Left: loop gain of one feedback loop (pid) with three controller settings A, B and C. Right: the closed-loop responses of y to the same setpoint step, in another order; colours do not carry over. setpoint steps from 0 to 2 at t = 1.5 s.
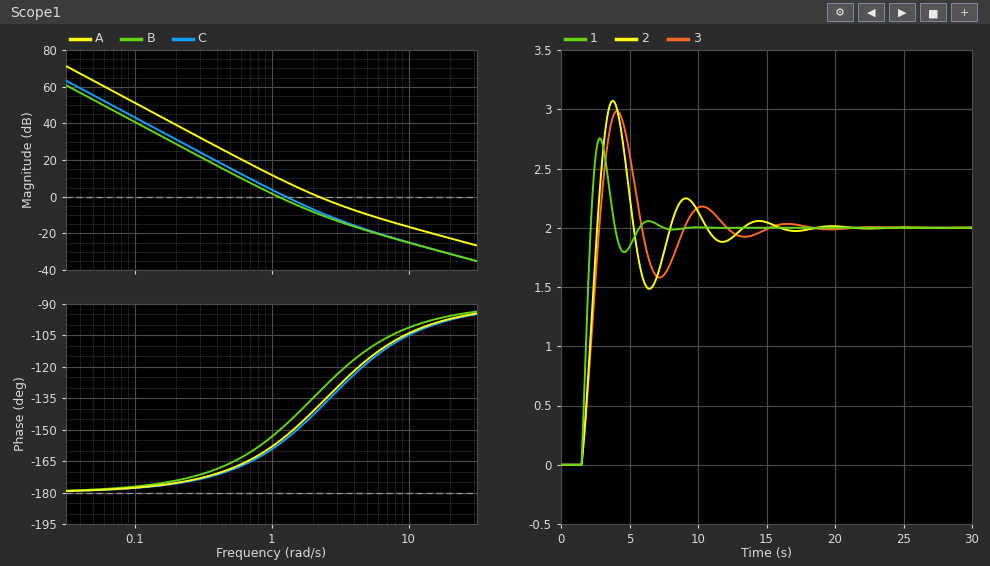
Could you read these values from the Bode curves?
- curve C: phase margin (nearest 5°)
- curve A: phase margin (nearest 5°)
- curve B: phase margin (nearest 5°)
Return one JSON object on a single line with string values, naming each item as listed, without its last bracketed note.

{"curve C: phase margin": "25°", "curve A: phase margin": "40°", "curve B: phase margin": "30°"}
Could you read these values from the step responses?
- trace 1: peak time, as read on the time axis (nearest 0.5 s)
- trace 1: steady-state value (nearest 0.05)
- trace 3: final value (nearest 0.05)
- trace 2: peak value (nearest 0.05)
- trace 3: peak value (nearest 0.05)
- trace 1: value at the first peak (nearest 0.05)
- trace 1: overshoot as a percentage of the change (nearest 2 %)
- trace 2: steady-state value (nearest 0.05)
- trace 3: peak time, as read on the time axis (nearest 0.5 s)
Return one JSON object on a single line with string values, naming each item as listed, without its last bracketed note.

{"trace 1: peak time, as read on the time axis": "3.0 s", "trace 1: steady-state value": "2.00", "trace 3: final value": "2.00", "trace 2: peak value": "3.05", "trace 3: peak value": "3.00", "trace 1: value at the first peak": "2.75", "trace 1: overshoot as a percentage of the change": "38 %", "trace 2: steady-state value": "2.00", "trace 3: peak time, as read on the time axis": "4.0 s"}
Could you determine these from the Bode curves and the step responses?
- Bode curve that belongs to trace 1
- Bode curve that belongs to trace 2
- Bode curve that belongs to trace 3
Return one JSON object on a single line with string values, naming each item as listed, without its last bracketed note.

{"Bode curve that belongs to trace 1": "A", "Bode curve that belongs to trace 2": "C", "Bode curve that belongs to trace 3": "B"}
